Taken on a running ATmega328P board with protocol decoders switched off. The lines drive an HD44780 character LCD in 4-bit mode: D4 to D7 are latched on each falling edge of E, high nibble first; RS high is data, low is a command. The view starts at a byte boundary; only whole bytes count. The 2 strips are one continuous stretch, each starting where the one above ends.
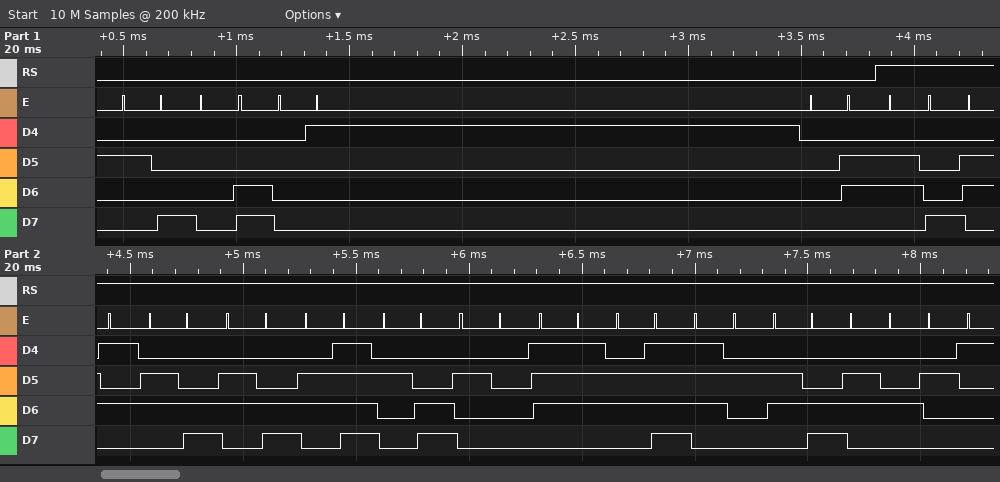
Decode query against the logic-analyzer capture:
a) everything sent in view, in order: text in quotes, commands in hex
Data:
0x28 0x0C 0x01 0x06 "hello, world!"
